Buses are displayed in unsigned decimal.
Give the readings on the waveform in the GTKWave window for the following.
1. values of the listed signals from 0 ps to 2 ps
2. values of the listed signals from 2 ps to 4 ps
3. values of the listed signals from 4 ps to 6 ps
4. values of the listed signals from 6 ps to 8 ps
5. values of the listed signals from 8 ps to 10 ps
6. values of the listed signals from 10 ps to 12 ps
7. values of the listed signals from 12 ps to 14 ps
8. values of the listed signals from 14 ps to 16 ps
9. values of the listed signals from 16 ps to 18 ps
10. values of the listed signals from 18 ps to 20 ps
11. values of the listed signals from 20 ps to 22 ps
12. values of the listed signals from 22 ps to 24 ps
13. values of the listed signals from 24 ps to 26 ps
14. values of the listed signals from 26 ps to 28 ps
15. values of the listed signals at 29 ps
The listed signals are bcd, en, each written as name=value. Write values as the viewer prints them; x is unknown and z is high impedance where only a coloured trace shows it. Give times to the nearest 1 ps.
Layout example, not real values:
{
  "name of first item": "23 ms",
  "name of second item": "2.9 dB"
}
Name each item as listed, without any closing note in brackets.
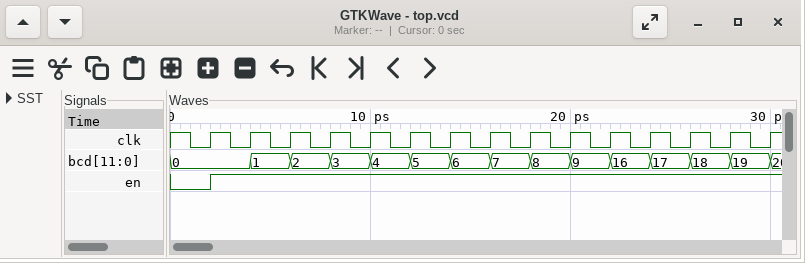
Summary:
{
  "values of the listed signals from 0 ps to 2 ps": "bcd=0, en=0",
  "values of the listed signals from 2 ps to 4 ps": "bcd=0, en=1",
  "values of the listed signals from 4 ps to 6 ps": "bcd=1, en=1",
  "values of the listed signals from 6 ps to 8 ps": "bcd=2, en=1",
  "values of the listed signals from 8 ps to 10 ps": "bcd=3, en=1",
  "values of the listed signals from 10 ps to 12 ps": "bcd=4, en=1",
  "values of the listed signals from 12 ps to 14 ps": "bcd=5, en=1",
  "values of the listed signals from 14 ps to 16 ps": "bcd=6, en=1",
  "values of the listed signals from 16 ps to 18 ps": "bcd=7, en=1",
  "values of the listed signals from 18 ps to 20 ps": "bcd=8, en=1",
  "values of the listed signals from 20 ps to 22 ps": "bcd=9, en=1",
  "values of the listed signals from 22 ps to 24 ps": "bcd=16, en=1",
  "values of the listed signals from 24 ps to 26 ps": "bcd=17, en=1",
  "values of the listed signals from 26 ps to 28 ps": "bcd=18, en=1",
  "values of the listed signals at 29 ps": "bcd=19, en=1"
}
